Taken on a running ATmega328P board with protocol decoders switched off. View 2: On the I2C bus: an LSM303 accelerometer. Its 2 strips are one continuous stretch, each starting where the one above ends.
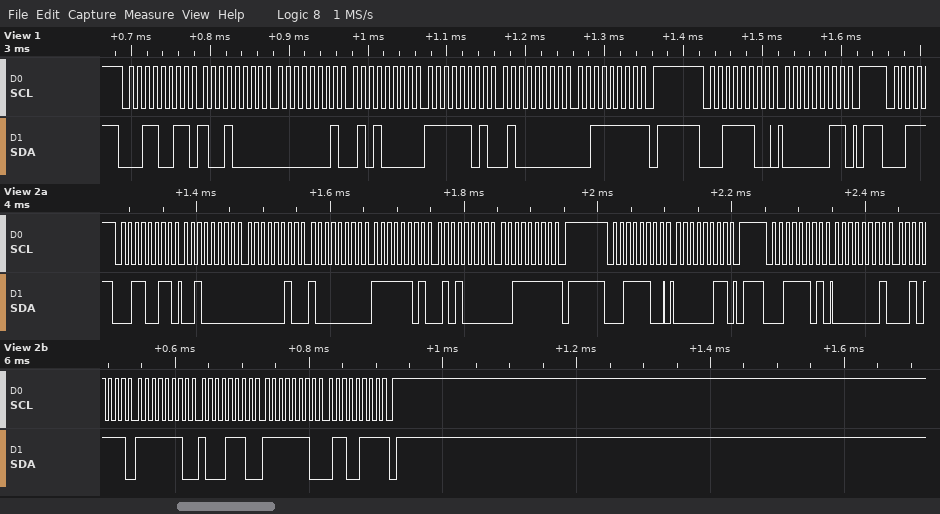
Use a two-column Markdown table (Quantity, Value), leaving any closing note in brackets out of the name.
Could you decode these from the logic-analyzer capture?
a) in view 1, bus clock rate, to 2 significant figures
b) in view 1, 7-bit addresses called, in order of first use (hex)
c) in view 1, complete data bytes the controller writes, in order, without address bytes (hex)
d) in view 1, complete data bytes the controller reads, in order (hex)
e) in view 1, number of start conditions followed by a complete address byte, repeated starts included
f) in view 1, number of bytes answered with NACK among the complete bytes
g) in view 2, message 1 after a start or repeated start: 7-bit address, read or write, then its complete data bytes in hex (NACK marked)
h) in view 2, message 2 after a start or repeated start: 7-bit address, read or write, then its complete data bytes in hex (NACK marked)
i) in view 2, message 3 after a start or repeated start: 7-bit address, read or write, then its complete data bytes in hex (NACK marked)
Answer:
| Quantity | Value |
|---|---|
| in view 1, bus clock rate, to 2 significant figures | 100 kHz |
| in view 1, 7-bit addresses called, in order of first use | 0x19 0x1E |
| in view 1, complete data bytes the controller writes, in order, without address bytes | 03 |
| in view 1, complete data bytes the controller reads, in order | 90 01 50 FD 40 3F |
| in view 1, number of start conditions followed by a complete address byte, repeated starts included | 2 |
| in view 1, number of bytes answered with NACK among the complete bytes | 1 |
| in view 2, message 1 after a start or repeated start: 7-bit address, read or write, then its complete data bytes in hex | 0x19 read: 20 02 80 FD 50 3F NACK |
| in view 2, message 2 after a start or repeated start: 7-bit address, read or write, then its complete data bytes in hex | 0x1E write: 03 |
| in view 2, message 3 after a start or repeated start: 7-bit address, read or write, then its complete data bytes in hex | 0x1E read: 01 2F FE 8E FE 67 NACK |
